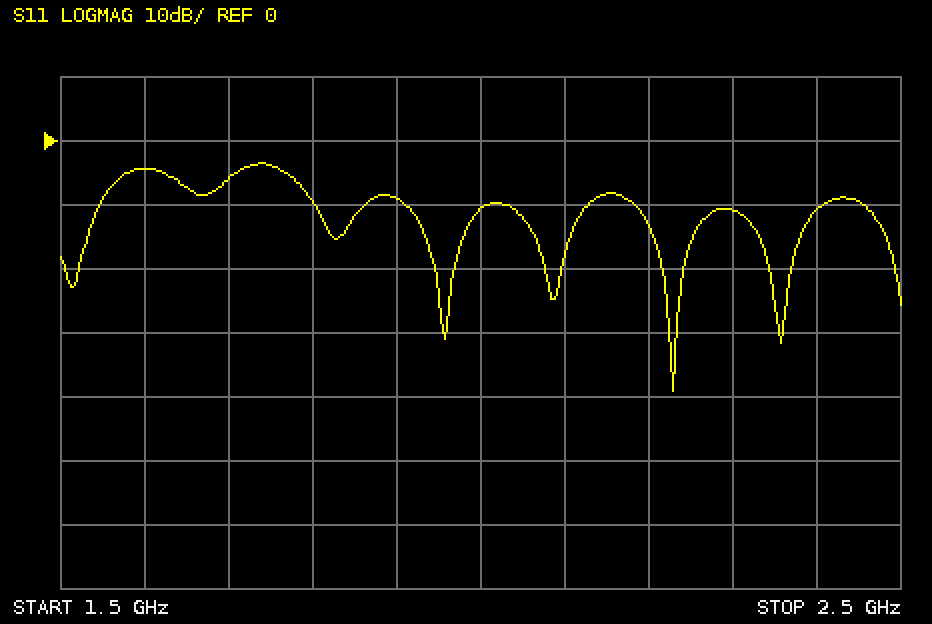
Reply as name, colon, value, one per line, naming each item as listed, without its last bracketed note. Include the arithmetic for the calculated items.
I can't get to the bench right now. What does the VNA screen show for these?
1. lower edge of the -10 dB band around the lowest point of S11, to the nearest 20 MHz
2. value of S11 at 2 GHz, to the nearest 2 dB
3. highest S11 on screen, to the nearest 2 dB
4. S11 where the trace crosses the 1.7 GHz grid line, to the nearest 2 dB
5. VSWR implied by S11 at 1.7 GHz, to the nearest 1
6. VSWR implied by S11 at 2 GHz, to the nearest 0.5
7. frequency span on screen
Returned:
lower edge of the -10 dB band around the lowest point of S11, to the nearest 20 MHz: 2.18 GHz
value of S11 at 2 GHz, to the nearest 2 dB: -10 dB
highest S11 on screen, to the nearest 2 dB: -4 dB
S11 where the trace crosses the 1.7 GHz grid line, to the nearest 2 dB: -6 dB
VSWR implied by S11 at 1.7 GHz, to the nearest 1: |Γ| = 10^(-6/20) = 0.5012; VSWR = (1 + 0.5012)/(1 − 0.5012) ≈ 3
VSWR implied by S11 at 2 GHz, to the nearest 0.5: |Γ| = 10^(-10/20) = 0.3162; VSWR = (1 + 0.3162)/(1 − 0.3162) ≈ 1.92, so 2.0 to the nearest 0.5
frequency span on screen: 1 GHz
